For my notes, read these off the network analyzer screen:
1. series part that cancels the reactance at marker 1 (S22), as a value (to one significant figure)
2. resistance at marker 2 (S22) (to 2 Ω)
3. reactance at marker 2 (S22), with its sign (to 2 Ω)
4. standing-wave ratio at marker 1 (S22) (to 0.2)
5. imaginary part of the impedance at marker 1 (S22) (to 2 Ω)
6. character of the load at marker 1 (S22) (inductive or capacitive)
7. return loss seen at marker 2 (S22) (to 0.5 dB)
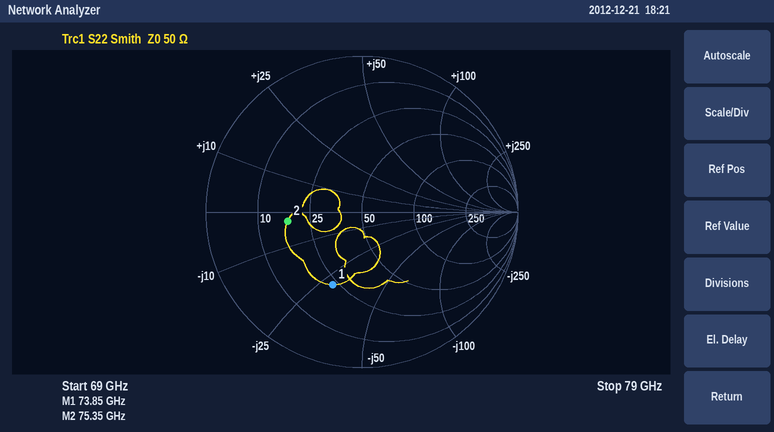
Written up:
60 pH
18 Ω
-2 Ω
3.0
-28 Ω
capacitive
6.5 dB
